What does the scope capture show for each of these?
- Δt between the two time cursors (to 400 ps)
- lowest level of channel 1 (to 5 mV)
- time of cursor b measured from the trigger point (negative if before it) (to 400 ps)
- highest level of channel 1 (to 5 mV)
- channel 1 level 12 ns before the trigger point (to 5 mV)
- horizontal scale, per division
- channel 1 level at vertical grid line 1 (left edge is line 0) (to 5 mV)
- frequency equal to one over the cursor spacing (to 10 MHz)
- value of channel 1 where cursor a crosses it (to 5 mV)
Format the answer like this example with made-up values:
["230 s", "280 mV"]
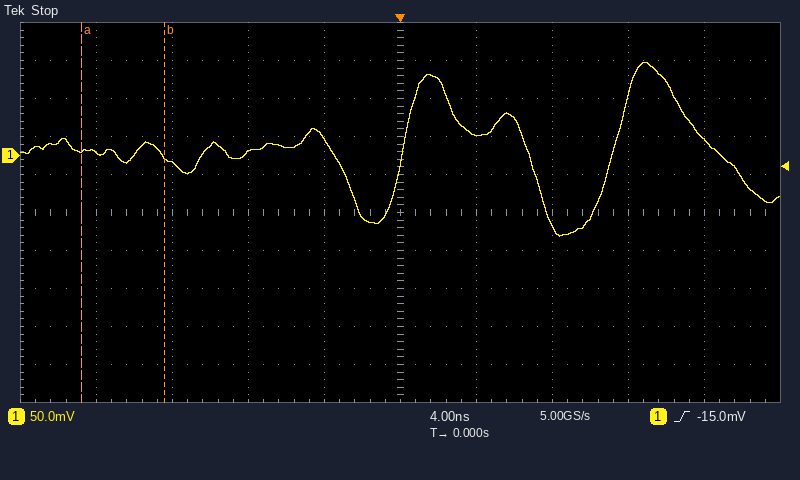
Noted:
["4.4 ns", "-105 mV", "-12.4 ns", "120 mV", "-10 mV", "4 ns", "5 mV", "230 MHz", "5 mV"]
